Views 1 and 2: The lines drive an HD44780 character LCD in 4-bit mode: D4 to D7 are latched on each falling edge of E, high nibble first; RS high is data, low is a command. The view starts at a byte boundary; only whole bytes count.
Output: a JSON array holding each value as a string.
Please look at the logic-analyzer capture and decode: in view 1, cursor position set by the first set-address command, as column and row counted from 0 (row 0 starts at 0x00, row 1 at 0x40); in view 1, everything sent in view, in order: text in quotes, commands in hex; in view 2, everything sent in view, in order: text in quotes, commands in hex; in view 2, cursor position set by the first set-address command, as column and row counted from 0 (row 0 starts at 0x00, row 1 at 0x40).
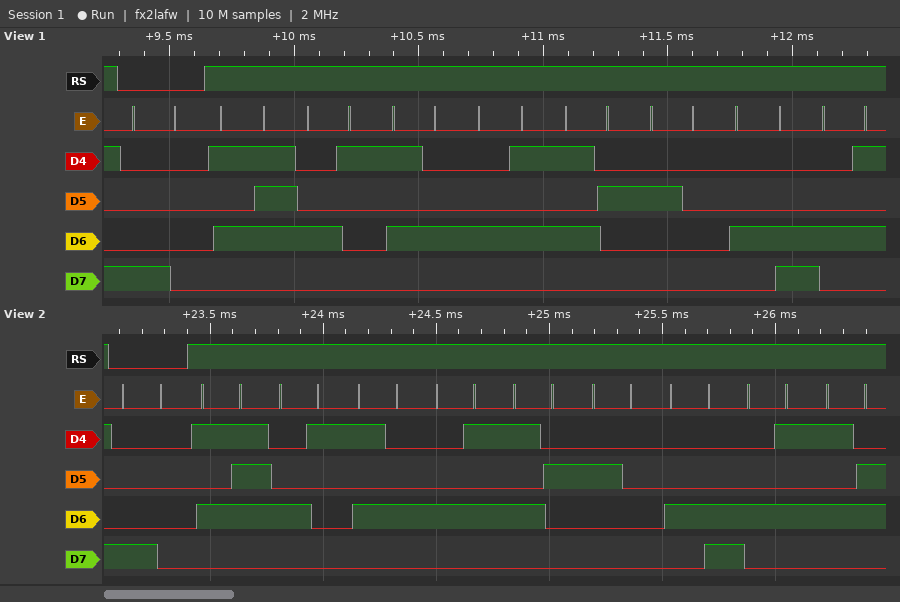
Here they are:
["column 0, row 0", "0x80 \"WATER LE\"", "0x80 \"WATER LEV\"", "column 0, row 0"]
